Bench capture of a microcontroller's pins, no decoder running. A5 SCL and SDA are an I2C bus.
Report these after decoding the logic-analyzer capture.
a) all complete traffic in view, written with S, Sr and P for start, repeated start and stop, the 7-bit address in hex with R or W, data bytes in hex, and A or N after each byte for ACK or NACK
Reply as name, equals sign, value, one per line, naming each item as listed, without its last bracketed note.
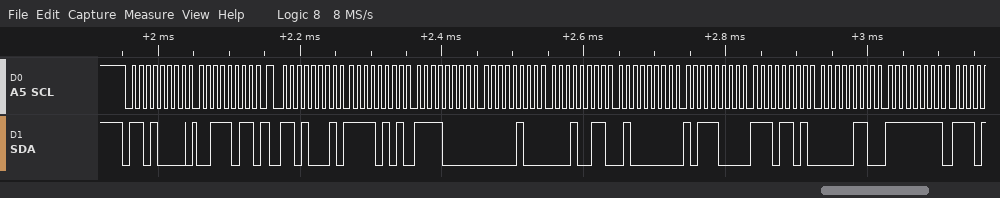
all complete traffic in view, written with S, Sr and P for start, repeated start and stop, the 7-bit address in hex with R or W, data bytes in hex, and A or N after each byte for ACK or NACK = S 68W A 3B A Sr 68R A F5 A F0 A 04 A 13 A 40 A B8 A ED A 06 A FF A
